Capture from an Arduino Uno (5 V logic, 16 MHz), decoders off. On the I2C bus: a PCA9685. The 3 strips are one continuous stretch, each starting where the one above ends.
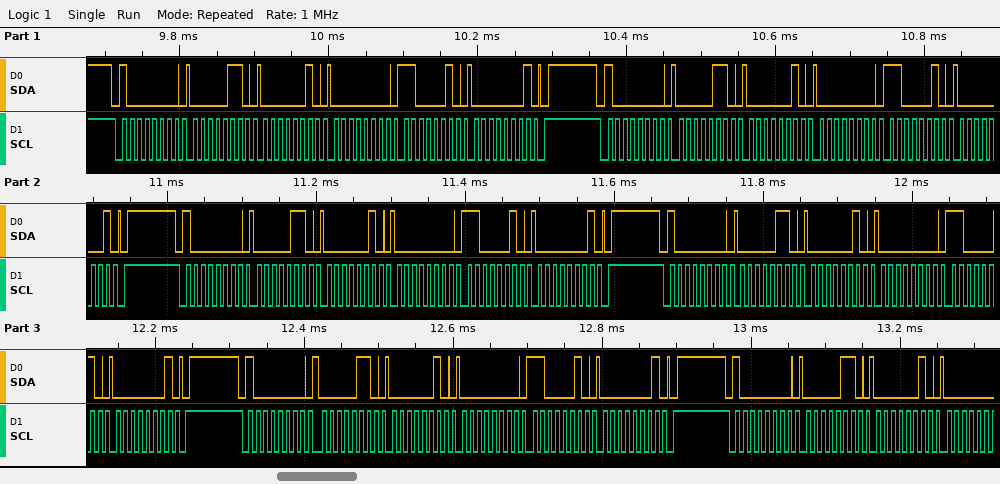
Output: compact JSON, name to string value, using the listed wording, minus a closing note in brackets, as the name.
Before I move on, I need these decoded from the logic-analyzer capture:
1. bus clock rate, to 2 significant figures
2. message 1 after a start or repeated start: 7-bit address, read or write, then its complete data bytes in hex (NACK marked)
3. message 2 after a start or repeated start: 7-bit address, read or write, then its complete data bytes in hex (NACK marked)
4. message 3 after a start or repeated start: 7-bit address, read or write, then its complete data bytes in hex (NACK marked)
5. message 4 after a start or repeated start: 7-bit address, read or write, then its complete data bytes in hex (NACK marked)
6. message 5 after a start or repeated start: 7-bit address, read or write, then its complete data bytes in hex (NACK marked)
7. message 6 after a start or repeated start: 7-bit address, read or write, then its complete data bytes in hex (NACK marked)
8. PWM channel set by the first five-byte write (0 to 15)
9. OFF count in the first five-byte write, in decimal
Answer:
{"bus clock rate, to 2 significant figures": "100 kHz", "message 1 after a start or repeated start: 7-bit address, read or write, then its complete data bytes in hex": "0x40 write: 06 02 00 C2 01", "message 2 after a start or repeated start: 7-bit address, read or write, then its complete data bytes in hex": "0x40 write: 06 02 00 C2 01", "message 3 after a start or repeated start: 7-bit address, read or write, then its complete data bytes in hex": "0x40 write: 06 02 00 C2 01", "message 4 after a start or repeated start: 7-bit address, read or write, then its complete data bytes in hex": "0x40 write: 06 02 00 C2 01", "message 5 after a start or repeated start: 7-bit address, read or write, then its complete data bytes in hex": "0x40 write: 06 02 00 C2 01", "message 6 after a start or repeated start: 7-bit address, read or write, then its complete data bytes in hex": "0x40 write: 06 02", "PWM channel set by the first five-byte write": "0", "OFF count in the first five-byte write, in decimal": "450"}
